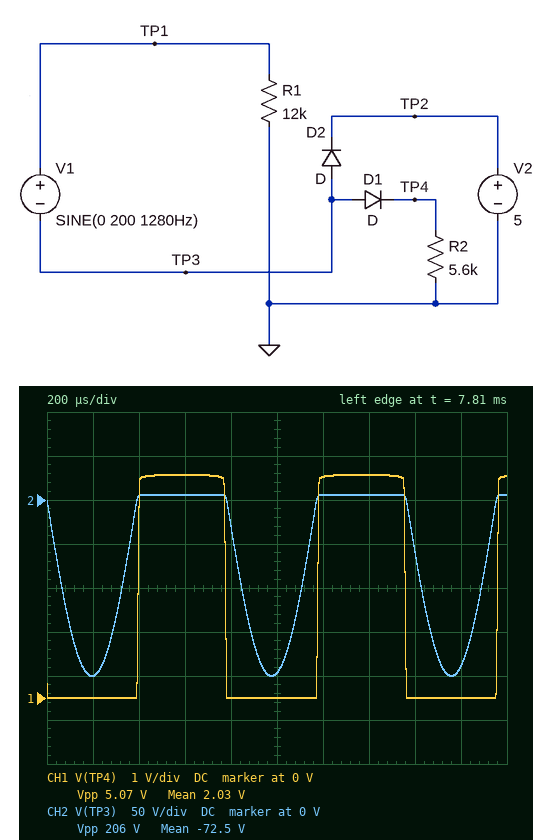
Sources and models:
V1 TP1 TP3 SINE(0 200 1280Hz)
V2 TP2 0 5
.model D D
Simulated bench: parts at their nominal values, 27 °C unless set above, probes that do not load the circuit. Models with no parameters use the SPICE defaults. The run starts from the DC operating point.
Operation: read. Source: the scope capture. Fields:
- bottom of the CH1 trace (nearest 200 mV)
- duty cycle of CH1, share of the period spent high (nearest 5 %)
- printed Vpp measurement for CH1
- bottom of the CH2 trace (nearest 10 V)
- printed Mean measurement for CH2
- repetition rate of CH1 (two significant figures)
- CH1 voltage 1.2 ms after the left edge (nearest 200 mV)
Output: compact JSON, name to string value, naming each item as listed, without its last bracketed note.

{"bottom of the CH1 trace": "0 V", "duty cycle of CH1, share of the period spent high": "50 %", "printed Vpp measurement for CH1": "5.07 V", "bottom of the CH2 trace": "-200 V", "printed Mean measurement for CH2": "-72.5 V", "repetition rate of CH1": "1.3 kHz", "CH1 voltage 1.2 ms after the left edge": "5.0 V"}
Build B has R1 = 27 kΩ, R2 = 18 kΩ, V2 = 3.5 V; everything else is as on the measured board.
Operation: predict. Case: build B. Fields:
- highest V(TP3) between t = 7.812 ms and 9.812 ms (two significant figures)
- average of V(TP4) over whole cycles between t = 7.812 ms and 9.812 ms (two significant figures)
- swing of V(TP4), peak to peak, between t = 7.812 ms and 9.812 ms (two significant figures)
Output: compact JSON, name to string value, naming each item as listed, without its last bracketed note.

{"highest V(TP3) between t = 7.812 ms and 9.812 ms": "4.2 V", "average of V(TP4) over whole cycles between t = 7.812 ms and 9.812 ms": "1.8 V", "swing of V(TP4), peak to peak, between t = 7.812 ms and 9.812 ms": "3.6 V"}
